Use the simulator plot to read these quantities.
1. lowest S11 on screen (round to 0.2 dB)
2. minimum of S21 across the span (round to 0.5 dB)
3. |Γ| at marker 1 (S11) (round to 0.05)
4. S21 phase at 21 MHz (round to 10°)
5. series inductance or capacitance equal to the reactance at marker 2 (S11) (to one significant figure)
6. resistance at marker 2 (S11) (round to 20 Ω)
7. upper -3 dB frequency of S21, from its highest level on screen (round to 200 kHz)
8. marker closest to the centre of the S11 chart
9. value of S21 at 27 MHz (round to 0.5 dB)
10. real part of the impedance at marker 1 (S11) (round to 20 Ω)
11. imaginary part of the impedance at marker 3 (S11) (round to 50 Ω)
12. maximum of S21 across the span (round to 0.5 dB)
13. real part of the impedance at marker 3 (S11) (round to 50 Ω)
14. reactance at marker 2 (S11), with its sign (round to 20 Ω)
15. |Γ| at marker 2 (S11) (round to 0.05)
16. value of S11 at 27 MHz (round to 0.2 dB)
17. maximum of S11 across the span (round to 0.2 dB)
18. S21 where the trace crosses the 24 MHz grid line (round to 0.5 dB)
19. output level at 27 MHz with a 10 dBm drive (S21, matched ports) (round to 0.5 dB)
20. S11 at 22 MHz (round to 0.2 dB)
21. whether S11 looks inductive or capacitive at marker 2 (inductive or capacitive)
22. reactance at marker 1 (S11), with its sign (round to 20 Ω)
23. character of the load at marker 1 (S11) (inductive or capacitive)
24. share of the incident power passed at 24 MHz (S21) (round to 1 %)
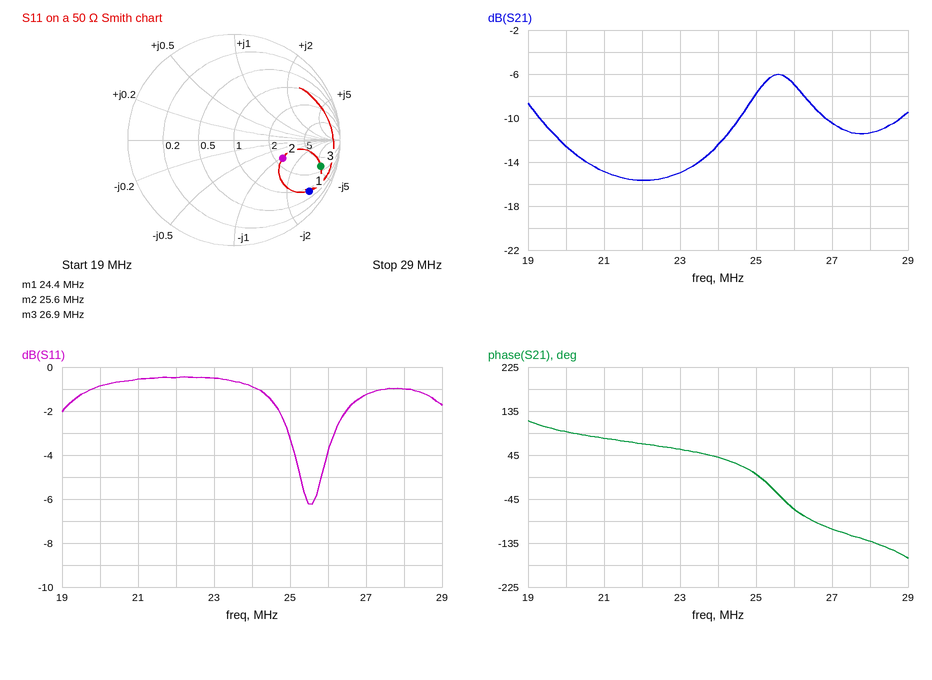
-6.2 dB
-15.5 dB
0.85
80°
100 pF
120 Ω
26.6 MHz
marker 2
-10.5 dB
40 Ω
-250 Ω
-6.0 dB
150 Ω
-60 Ω
0.50
-1.2 dB
-0.4 dB
-12.5 dB
-0.5 dBm
-0.4 dB
capacitive
-160 Ω
capacitive
6 %
